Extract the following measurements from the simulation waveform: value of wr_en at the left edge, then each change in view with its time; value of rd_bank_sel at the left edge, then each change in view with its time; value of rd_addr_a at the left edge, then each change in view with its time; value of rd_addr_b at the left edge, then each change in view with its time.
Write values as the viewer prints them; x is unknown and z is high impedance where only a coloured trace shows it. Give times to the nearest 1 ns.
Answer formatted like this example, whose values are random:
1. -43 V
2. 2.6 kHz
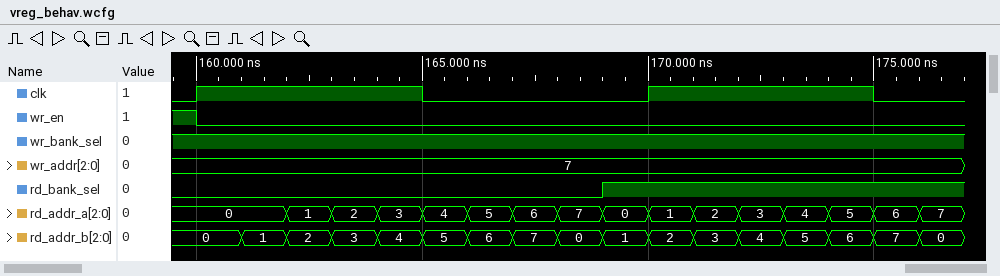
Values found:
1. 1, 0 at 160 ns
2. 0, 1 at 169 ns
3. 0, 1 at 162 ns, 2 at 163 ns, 3 at 164 ns, 4 at 165 ns, 5 at 166 ns, 6 at 167 ns, 7 at 168 ns, 0 at 169 ns, 1 at 170 ns, 2 at 171 ns, 3 at 172 ns, 4 at 173 ns, 5 at 174 ns, 6 at 175 ns, 7 at 176 ns
4. 0, 1 at 161 ns, 2 at 162 ns, 3 at 163 ns, 4 at 164 ns, 5 at 165 ns, 6 at 166 ns, 7 at 167 ns, 0 at 168 ns, 1 at 169 ns, 2 at 170 ns, 3 at 171 ns, 4 at 172 ns, 5 at 173 ns, 6 at 174 ns, 7 at 175 ns, 0 at 176 ns
